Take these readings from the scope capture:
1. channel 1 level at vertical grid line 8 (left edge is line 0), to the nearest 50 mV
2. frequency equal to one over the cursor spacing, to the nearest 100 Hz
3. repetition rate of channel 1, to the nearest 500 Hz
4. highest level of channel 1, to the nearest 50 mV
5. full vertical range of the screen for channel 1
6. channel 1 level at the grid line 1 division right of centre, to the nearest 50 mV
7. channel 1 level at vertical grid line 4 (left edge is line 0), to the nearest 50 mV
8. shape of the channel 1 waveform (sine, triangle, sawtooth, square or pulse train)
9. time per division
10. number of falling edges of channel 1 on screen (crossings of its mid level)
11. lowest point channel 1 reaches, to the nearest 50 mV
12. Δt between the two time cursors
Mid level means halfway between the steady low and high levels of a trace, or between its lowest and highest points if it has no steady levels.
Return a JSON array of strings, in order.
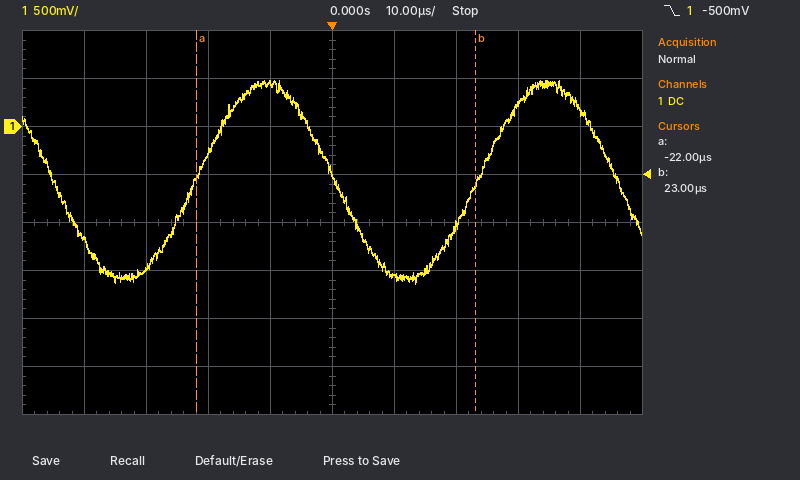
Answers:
["250 mV", "22.2 kHz", "22.0 kHz", "500 mV", "4 V", "-1.55 V", "450 mV", "sine", "10 µs", "3", "-1.65 V", "45 µs"]
